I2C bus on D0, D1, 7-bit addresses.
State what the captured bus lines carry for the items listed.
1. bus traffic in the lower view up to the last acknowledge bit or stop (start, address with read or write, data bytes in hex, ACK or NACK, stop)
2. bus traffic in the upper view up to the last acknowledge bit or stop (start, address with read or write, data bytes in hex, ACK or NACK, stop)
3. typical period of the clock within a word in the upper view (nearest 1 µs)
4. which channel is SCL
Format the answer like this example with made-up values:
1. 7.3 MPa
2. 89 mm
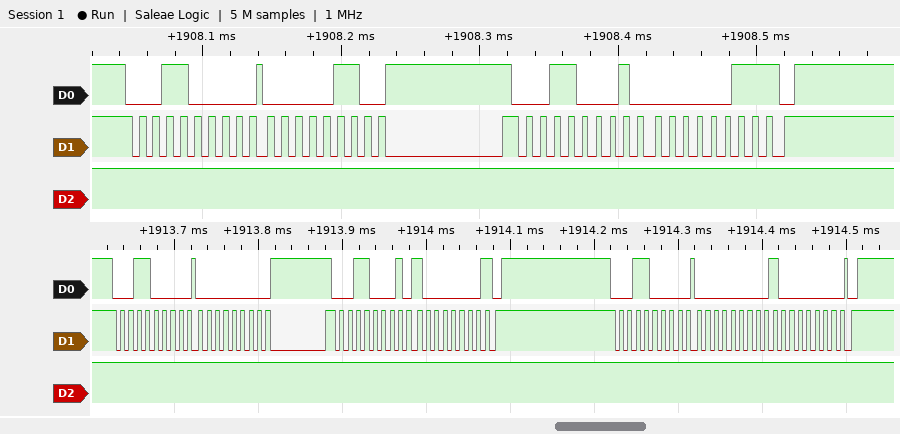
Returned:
1. start, address 18 write ACK, 00 ACK, repeated start, address 18 read ACK, 80 NACK, stop, start, address 18 write ACK, 00 ACK, 80 ACK, stop
2. start, address 18 write ACK, 06 ACK, repeated start, address 18 read ACK, 03 NACK, stop
3. 10 µs
4. D1
